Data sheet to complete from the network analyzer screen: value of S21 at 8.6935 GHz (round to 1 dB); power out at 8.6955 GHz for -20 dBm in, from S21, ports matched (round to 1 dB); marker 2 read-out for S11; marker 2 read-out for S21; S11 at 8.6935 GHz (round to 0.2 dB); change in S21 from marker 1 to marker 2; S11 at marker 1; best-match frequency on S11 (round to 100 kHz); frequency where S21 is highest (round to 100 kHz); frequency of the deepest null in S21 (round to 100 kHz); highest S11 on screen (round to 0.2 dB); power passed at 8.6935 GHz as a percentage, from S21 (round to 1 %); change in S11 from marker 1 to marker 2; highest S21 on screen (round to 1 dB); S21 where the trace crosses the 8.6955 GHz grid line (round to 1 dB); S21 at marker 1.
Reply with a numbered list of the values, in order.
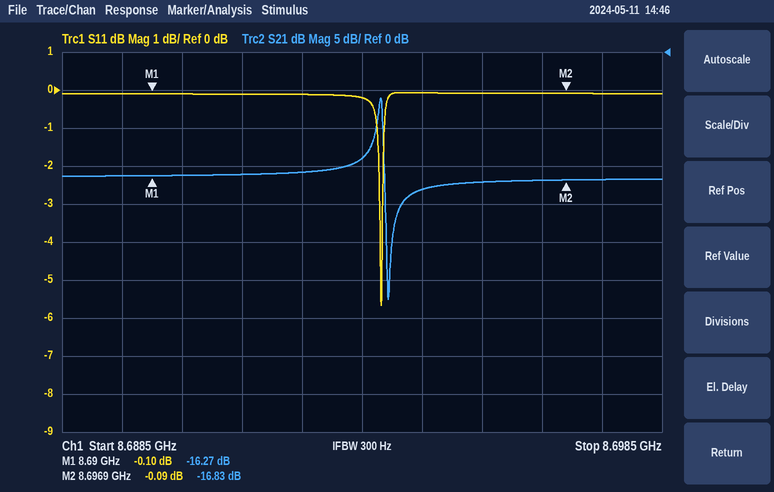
1. -14 dB
2. -37 dBm
3. -0.09 dB
4. -16.83 dB
5. -0.2 dB
6. -0.56 dB
7. -0.10 dB
8. 8.6938 GHz
9. 8.6938 GHz
10. 8.6939 GHz
11. 0.0 dB
12. 4 %
13. 0.01 dB
14. -6 dB
15. -17 dB
16. -16.27 dB
